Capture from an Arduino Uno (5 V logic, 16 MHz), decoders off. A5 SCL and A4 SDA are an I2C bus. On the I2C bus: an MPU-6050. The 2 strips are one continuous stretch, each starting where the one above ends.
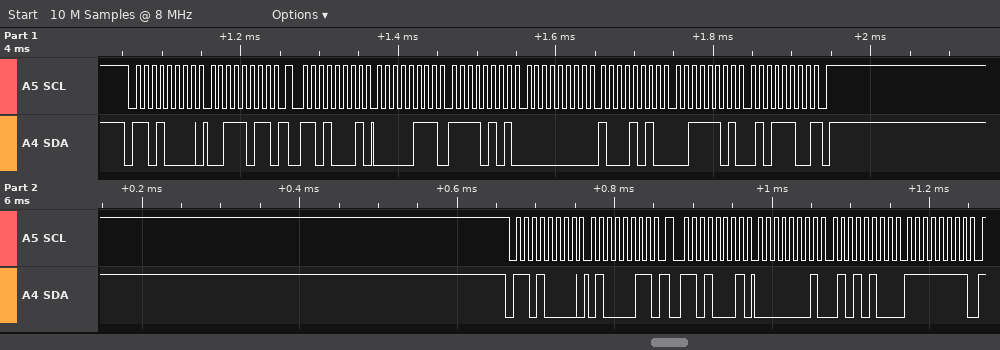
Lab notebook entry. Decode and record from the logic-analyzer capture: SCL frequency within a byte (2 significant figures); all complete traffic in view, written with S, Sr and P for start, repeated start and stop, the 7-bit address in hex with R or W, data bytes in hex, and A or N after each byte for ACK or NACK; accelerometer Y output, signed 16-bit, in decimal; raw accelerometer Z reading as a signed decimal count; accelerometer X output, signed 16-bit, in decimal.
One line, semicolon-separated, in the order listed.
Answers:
100 kHz; S 68W A 3B A Sr 68R A 07 A F5 A 00 A 8A A 3D A 5C N P S 68W A 43 A Sr 68R A 01 A 54 A FF A; 138; 15708; 2037
